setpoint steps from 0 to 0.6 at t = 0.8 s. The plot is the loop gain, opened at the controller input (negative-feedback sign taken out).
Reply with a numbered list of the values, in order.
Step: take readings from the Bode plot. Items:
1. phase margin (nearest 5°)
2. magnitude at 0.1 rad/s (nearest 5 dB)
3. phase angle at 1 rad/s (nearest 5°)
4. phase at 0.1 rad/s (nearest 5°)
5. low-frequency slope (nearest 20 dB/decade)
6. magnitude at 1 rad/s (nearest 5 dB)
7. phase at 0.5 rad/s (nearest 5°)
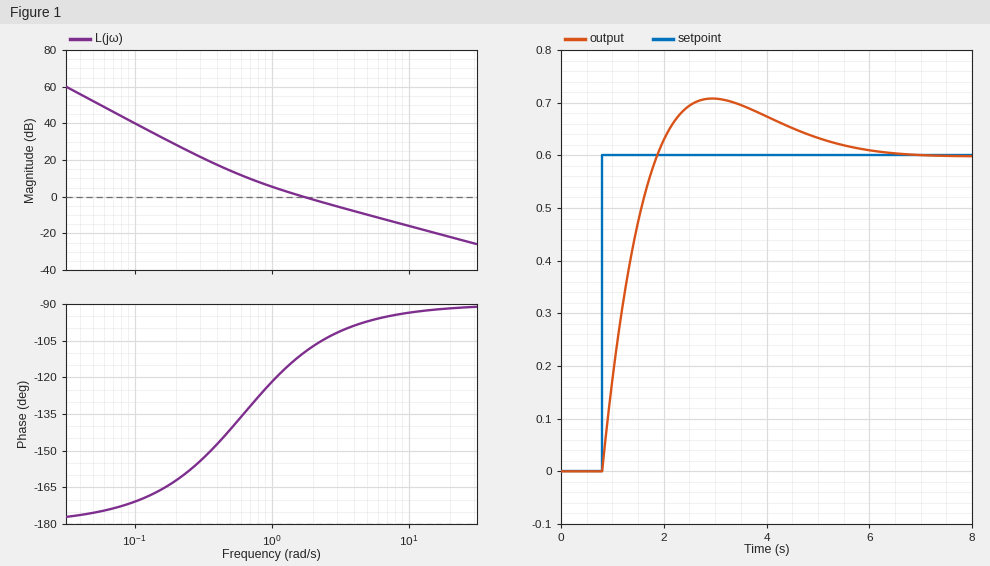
1. 70°
2. 40 dB
3. -120°
4. -170°
5. -40 dB/decade
6. 5 dB
7. -140°
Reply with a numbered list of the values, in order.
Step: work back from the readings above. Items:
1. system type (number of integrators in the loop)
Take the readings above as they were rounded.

1. 2
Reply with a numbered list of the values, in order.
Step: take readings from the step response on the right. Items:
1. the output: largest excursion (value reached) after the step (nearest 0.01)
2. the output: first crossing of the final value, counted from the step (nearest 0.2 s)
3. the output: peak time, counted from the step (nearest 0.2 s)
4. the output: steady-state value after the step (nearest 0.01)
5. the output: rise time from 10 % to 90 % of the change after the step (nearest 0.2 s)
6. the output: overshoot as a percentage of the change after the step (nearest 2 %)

1. 0.71
2. 1.0 s
3. 2.2 s
4. 0.60
5. 0.8 s
6. 18 %
